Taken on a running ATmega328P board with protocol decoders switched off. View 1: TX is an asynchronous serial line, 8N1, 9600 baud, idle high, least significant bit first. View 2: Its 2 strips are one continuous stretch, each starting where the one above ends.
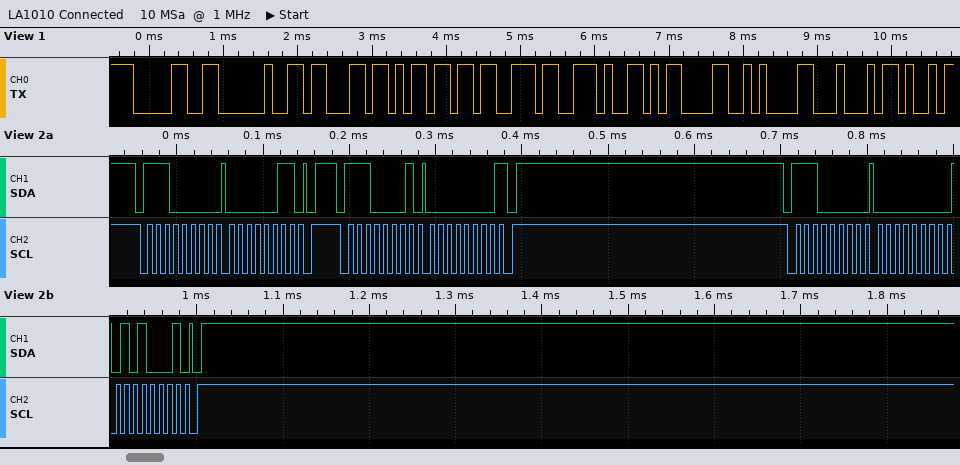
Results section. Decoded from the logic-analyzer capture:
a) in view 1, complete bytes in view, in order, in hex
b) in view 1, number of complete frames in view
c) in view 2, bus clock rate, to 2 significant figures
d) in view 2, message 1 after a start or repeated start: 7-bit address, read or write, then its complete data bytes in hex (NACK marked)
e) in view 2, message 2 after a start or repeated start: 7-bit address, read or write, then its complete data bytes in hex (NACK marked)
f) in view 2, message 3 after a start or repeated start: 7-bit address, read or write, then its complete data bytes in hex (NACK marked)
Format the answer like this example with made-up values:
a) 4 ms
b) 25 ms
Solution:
a) 30 20 63 6D 73 2E 0D 0A 44
b) 9
c) 100 kHz
d) 0x70 write: 03
e) 0x70 read: 00 NACK
f) 0x70 write: 00 51
